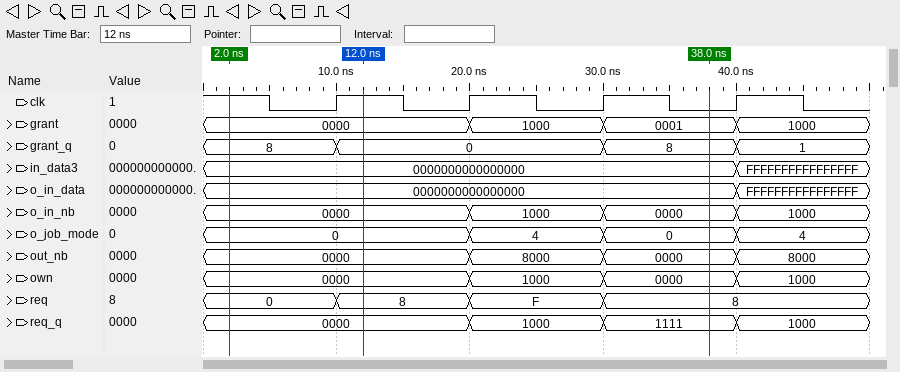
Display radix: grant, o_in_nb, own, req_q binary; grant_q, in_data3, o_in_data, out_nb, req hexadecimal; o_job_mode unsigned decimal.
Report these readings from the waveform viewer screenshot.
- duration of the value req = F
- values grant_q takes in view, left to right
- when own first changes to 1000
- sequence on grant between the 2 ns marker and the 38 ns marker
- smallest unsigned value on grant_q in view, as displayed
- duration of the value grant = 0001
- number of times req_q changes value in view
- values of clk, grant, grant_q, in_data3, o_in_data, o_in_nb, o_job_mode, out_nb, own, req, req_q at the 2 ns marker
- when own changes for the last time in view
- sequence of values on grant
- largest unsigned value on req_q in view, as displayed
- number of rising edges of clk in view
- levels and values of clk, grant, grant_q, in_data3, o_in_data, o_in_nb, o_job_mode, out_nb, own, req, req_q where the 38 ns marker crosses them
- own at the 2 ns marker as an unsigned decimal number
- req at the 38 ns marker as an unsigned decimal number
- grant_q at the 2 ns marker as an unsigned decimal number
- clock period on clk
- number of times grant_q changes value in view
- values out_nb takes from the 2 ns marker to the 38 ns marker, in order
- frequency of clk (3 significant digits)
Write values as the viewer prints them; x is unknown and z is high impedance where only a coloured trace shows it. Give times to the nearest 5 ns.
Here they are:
10 ns
8, 0, 8, 1
20 ns
0000, 1000, 0001
0
10 ns
3
clk=1, grant=0000, grant_q=8, in_data3=0000000000000000, o_in_data=0000000000000000, o_in_nb=0000, o_job_mode=0, out_nb=0000, own=0000, req=0, req_q=0000
40 ns
0000, 1000, 0001, 1000
1111
4
clk=0, grant=0001, grant_q=8, in_data3=0000000000000000, o_in_data=0000000000000000, o_in_nb=0000, o_job_mode=0, out_nb=0000, own=0000, req=8, req_q=1111
0
8
8
10 ns
3
0000, 8000, 0000
100 MHz
